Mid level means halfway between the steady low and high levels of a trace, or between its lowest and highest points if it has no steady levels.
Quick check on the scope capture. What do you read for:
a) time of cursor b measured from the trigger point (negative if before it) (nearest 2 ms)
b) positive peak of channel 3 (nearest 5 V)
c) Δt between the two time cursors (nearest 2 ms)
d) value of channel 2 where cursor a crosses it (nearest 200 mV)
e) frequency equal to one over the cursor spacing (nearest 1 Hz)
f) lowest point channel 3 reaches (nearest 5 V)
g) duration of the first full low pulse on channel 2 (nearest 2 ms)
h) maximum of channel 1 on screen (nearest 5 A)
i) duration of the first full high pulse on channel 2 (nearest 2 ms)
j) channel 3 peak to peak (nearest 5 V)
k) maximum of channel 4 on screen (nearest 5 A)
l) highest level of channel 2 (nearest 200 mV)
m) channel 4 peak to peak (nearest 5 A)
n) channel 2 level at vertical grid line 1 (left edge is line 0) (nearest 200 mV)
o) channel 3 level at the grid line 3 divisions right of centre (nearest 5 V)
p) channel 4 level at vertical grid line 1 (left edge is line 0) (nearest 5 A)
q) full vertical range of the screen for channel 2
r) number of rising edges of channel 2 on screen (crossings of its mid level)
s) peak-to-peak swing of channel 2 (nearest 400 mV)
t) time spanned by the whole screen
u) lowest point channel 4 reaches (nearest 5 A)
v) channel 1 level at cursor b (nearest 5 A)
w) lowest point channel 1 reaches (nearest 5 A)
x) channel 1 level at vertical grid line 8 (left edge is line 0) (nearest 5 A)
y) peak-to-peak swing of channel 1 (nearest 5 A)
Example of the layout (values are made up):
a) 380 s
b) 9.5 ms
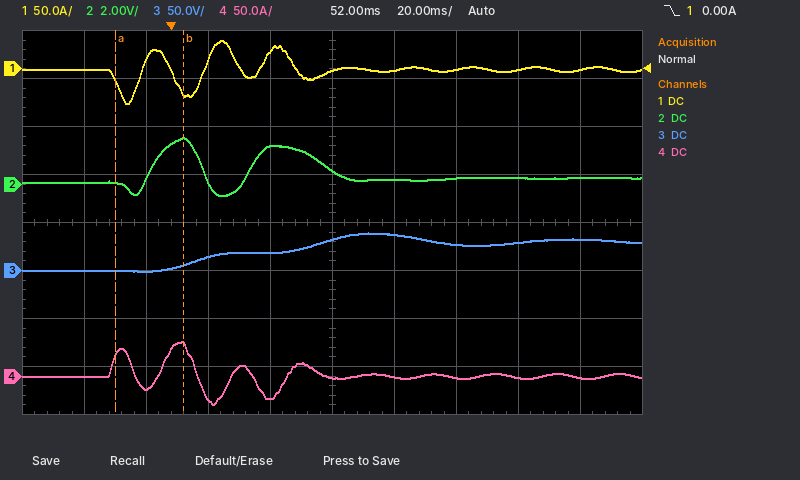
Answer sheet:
a) +4 ms
b) 40 V
c) 22 ms
d) 0.0 V
e) 45 Hz
f) 0 V
g) 16 ms
h) 30 A
i) 16 ms
j) 40 V
k) 35 A
l) 2.0 V
m) 65 A
n) 0.0 V
o) 30 V
p) 0 A
q) 16 V
r) 2
s) 2.4 V
t) 200 ms
u) -30 A
v) -25 A
w) -35 A
x) 0 A
y) 65 A
